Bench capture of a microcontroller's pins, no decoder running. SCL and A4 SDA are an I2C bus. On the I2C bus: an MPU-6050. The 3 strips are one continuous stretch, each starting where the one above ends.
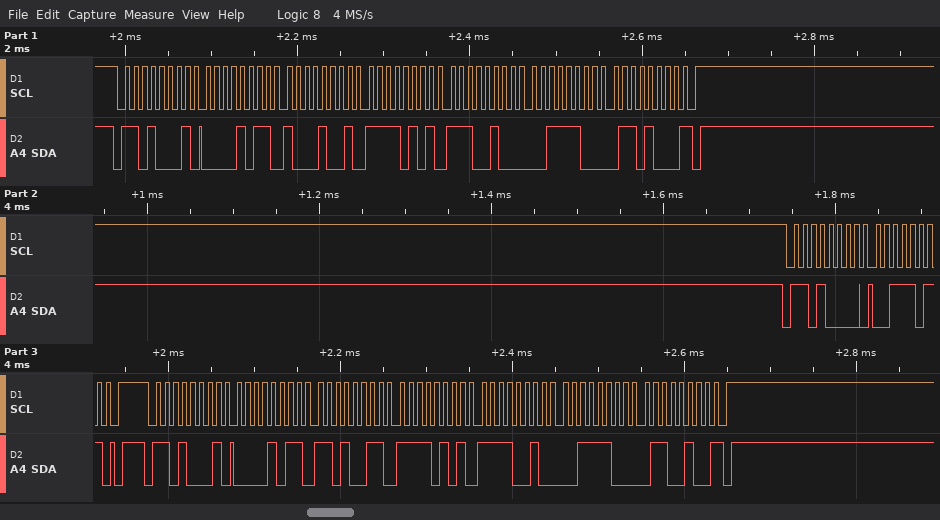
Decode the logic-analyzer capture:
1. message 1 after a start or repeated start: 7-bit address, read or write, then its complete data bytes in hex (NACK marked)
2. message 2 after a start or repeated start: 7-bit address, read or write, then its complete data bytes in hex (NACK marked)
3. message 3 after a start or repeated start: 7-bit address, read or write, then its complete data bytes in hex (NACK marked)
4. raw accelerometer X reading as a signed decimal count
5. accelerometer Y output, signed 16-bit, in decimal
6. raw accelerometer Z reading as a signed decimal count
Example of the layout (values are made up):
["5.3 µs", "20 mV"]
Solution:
["0x68 read: 0B 89 F5 E4 3C 68 NACK", "0x68 write: 3B", "0x68 read: 0B D3 F5 F2 3C 64 NACK", "3027", "-2574", "15460"]
